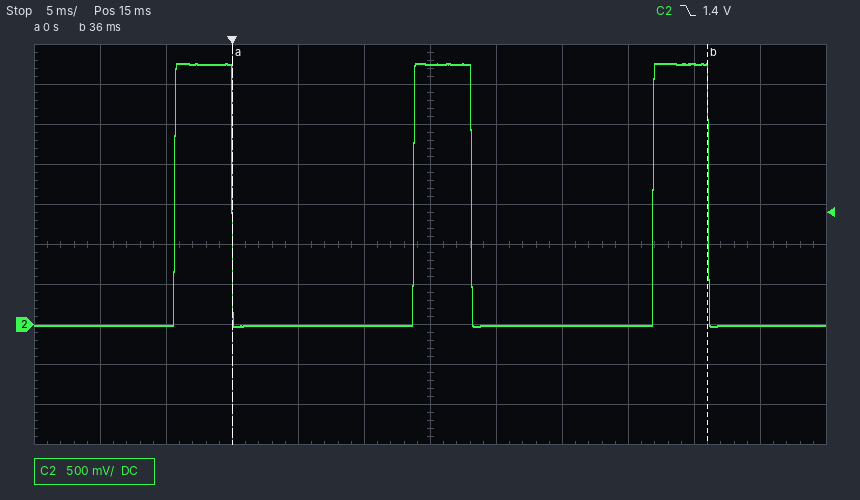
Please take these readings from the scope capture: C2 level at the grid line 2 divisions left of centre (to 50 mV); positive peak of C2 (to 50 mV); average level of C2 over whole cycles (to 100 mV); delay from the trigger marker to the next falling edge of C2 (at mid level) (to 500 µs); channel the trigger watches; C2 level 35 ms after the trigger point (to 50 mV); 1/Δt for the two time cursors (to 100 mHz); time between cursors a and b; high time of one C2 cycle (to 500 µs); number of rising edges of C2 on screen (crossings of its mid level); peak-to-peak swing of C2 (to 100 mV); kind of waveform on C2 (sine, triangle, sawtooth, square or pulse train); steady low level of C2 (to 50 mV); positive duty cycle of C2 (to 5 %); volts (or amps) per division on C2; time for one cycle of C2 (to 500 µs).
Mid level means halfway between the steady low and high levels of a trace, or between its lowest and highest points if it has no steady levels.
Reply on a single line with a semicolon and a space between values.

0 mV; 3.25 V; 800 mV; 18.0 ms; C2; 3.25 V; 27.8 Hz; 36.0 ms; 4.5 ms; 3; 3.30 V; pulse train; 0 mV; 25 %; 500 mV; 18.0 ms
